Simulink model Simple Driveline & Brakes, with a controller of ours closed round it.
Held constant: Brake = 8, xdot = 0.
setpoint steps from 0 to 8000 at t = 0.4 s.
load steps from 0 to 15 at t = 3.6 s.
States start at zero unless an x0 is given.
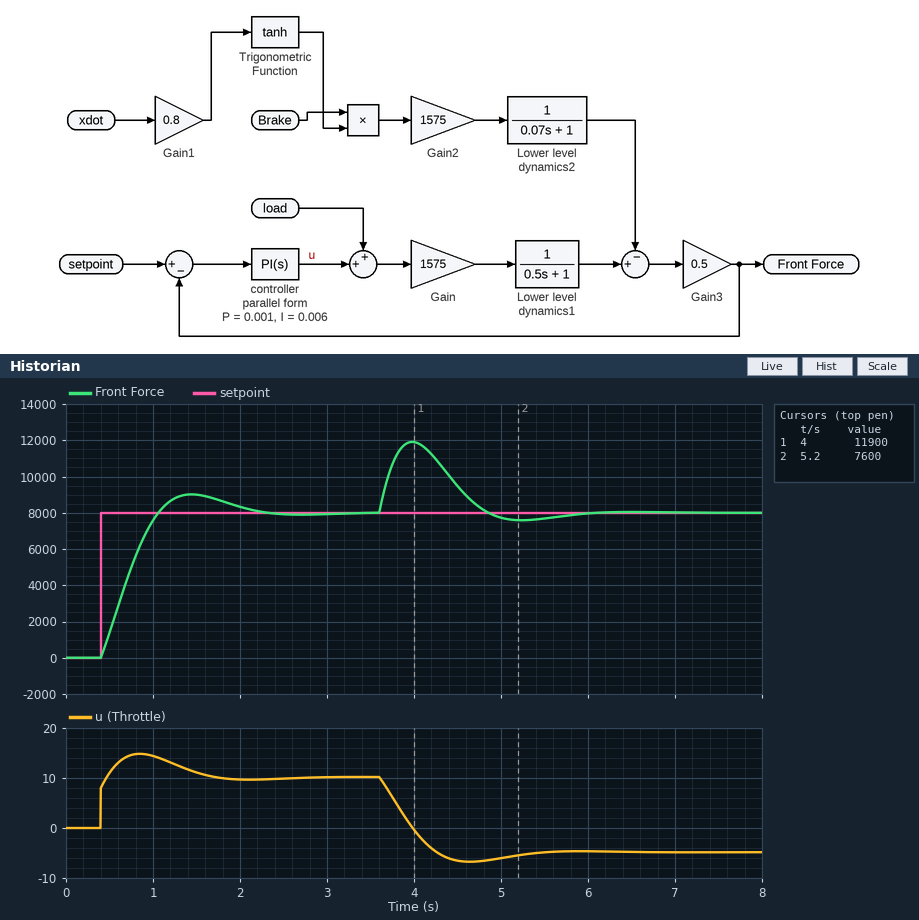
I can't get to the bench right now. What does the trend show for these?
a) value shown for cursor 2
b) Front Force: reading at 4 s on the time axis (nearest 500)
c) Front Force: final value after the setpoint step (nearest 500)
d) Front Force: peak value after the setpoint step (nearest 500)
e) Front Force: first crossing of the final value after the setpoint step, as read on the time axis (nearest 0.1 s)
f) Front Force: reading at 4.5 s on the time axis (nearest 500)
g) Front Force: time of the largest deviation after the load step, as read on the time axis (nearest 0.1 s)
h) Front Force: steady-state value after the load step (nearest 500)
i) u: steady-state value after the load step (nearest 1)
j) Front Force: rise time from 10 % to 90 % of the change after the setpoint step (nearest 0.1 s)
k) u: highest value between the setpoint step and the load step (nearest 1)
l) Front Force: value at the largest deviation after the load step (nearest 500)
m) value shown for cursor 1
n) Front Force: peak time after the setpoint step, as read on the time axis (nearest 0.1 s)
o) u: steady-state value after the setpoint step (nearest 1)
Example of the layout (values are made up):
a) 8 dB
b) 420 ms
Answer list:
a) 7600
b) 12000
c) 8000
d) 9000
e) 1.1 s
f) 9500
g) 4.0 s
h) 8000
i) -5
j) 0.5 s
k) 15
l) 12000
m) 11900
n) 1.4 s
o) 10
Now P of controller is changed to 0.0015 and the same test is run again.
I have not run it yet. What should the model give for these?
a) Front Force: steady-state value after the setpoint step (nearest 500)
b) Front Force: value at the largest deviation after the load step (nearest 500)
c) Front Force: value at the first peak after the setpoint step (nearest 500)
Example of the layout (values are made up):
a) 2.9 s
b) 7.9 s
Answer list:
a) 8000
b) 11500
c) 8500
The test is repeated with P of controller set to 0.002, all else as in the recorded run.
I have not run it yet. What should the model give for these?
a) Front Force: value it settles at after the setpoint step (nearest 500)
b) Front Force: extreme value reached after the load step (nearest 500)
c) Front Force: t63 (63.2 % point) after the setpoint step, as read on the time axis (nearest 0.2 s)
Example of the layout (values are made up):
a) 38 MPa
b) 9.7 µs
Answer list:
a) 8000
b) 11000
c) 0.6 s
